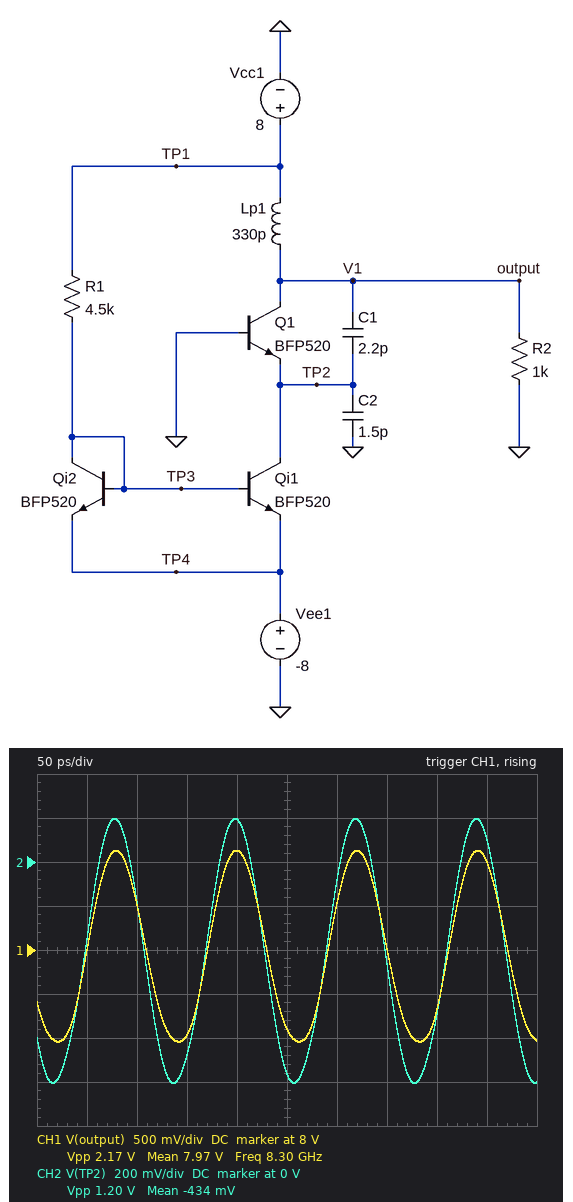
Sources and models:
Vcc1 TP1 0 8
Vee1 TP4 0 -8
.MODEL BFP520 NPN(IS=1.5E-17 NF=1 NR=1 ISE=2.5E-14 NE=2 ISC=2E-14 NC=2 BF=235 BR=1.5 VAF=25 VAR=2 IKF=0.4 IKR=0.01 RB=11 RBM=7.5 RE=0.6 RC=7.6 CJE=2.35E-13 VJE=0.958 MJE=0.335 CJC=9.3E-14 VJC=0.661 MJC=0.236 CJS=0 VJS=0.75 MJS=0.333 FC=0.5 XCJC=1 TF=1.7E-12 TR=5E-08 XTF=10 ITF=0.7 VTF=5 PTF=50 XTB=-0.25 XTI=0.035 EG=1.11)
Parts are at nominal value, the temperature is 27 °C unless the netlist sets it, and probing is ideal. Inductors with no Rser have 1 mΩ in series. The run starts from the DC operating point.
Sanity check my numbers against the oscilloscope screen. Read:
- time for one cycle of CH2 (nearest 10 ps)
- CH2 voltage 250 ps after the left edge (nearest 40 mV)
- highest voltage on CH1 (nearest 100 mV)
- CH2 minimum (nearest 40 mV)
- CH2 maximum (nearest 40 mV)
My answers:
120 ps
-960 mV
9.1 V
-1.00 V
200 mV
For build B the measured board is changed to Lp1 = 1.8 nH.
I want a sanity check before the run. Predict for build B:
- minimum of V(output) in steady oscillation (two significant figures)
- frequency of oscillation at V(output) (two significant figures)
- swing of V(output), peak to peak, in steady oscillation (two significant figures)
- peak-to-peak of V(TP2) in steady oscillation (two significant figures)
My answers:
4.6 V
3.6 GHz
6.8 V
3.7 V
